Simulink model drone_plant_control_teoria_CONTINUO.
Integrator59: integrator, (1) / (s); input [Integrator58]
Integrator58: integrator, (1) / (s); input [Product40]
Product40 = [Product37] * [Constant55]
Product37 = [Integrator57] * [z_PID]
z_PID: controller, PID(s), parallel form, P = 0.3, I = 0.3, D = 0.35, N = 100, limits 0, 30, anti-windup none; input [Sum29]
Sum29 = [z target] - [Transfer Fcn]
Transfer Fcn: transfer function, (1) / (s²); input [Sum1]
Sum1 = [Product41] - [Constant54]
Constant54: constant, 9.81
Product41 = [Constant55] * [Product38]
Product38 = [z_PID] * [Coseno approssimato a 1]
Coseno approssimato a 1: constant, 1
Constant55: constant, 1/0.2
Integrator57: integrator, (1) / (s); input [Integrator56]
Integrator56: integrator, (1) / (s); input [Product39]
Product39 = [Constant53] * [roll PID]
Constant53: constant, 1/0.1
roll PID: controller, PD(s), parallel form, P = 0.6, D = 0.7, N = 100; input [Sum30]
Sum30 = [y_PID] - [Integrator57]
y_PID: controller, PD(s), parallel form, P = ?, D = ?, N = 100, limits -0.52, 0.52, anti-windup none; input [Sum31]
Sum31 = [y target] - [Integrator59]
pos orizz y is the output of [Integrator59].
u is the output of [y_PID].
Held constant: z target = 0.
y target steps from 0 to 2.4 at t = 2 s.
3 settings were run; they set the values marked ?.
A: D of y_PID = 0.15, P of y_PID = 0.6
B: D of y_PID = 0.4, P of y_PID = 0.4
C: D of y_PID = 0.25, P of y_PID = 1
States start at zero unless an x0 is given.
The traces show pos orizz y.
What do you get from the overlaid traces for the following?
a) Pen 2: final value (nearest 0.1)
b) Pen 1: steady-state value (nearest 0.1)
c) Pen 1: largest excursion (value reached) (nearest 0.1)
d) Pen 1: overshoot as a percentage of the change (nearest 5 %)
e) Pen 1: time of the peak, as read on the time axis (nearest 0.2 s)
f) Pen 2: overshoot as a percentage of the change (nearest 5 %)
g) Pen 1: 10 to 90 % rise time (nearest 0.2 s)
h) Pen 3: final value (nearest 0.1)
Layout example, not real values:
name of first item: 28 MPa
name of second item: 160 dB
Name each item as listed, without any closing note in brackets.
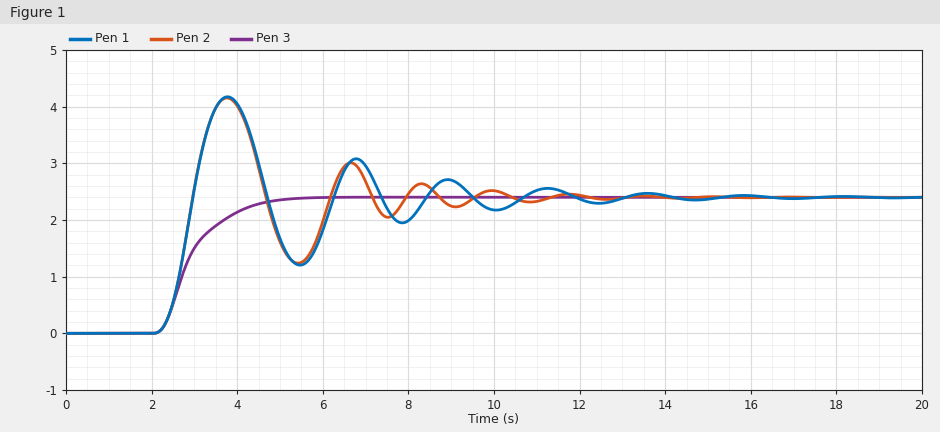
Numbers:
Pen 2: final value: 2.4
Pen 1: steady-state value: 2.4
Pen 1: largest excursion (value reached): 4.2
Pen 1: overshoot as a percentage of the change: 75 %
Pen 1: time of the peak, as read on the time axis: 3.8 s
Pen 2: overshoot as a percentage of the change: 75 %
Pen 1: 10 to 90 % rise time: 0.6 s
Pen 3: final value: 2.4
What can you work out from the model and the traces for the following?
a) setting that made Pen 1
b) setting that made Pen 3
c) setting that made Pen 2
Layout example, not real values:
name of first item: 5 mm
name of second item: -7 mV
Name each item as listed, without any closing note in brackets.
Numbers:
setting that made Pen 1: A
setting that made Pen 3: B
setting that made Pen 2: C
